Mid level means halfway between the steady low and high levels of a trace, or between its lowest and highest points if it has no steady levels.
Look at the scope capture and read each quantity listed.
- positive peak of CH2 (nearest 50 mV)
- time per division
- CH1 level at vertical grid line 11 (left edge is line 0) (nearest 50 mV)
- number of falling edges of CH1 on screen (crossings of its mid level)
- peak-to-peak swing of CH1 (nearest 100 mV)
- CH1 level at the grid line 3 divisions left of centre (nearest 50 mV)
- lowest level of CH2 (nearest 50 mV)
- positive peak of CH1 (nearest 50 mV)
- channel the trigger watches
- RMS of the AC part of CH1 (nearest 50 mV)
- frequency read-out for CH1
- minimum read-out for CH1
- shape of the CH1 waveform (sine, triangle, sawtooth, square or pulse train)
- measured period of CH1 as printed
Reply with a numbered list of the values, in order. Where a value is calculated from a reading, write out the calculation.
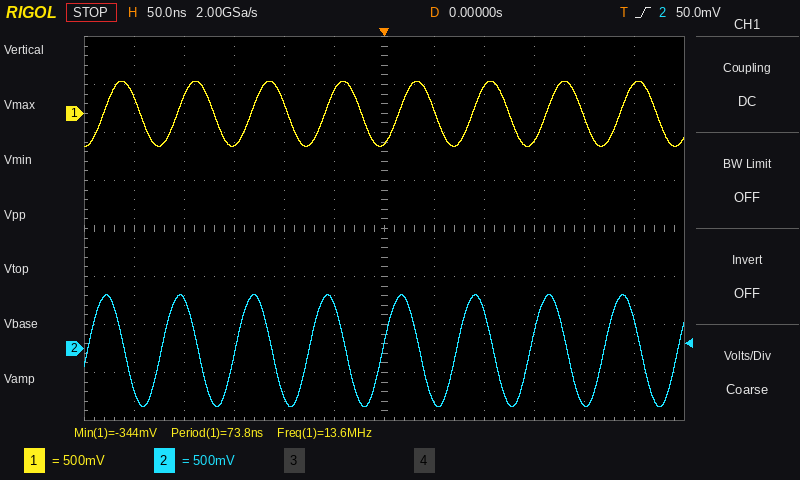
1. 550 mV
2. 50 ns
3. 300 mV
4. 8
5. 700 mV
6. -350 mV
7. -600 mV
8. 350 mV
9. CH2
10. 700 mV / (2√2) ≈ 247 mV, so 250 mV to the nearest 50 mV
11. 13.6 MHz
12. -344 mV
13. sine
14. 73.8 ns
